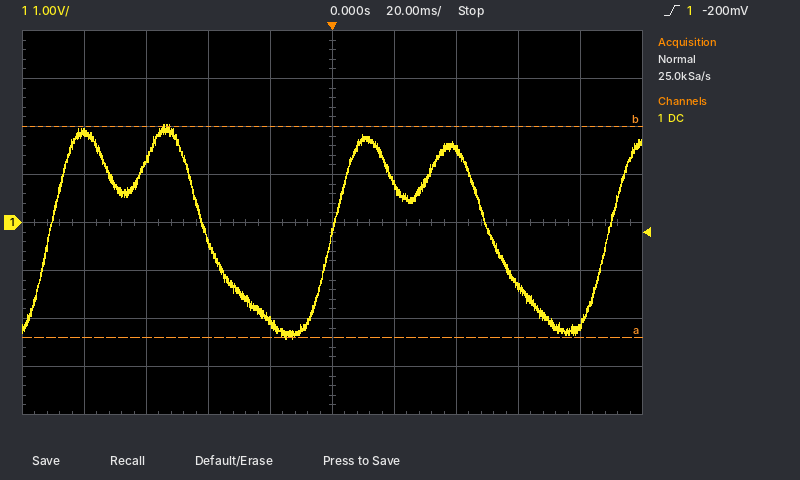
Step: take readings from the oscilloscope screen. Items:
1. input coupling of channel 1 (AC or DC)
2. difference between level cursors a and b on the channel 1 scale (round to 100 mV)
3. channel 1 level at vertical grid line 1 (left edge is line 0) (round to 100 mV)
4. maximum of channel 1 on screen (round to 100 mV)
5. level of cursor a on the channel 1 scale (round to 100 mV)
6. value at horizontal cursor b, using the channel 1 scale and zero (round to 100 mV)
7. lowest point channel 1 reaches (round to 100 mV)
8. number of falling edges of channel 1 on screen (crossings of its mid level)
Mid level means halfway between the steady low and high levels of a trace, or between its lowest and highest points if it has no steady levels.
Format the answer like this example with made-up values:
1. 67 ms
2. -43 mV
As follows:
1. DC
2. 4.4 V
3. 1.9 V
4. 2.0 V
5. -2.4 V
6. 2.0 V
7. -2.4 V
8. 2
